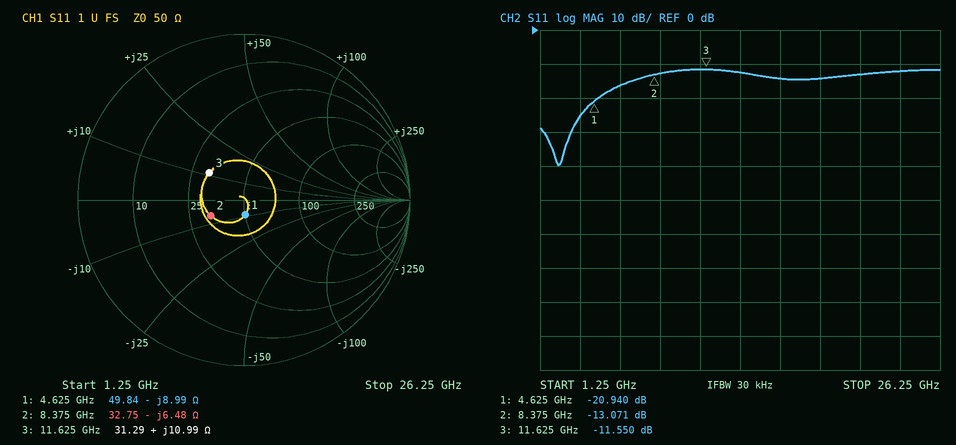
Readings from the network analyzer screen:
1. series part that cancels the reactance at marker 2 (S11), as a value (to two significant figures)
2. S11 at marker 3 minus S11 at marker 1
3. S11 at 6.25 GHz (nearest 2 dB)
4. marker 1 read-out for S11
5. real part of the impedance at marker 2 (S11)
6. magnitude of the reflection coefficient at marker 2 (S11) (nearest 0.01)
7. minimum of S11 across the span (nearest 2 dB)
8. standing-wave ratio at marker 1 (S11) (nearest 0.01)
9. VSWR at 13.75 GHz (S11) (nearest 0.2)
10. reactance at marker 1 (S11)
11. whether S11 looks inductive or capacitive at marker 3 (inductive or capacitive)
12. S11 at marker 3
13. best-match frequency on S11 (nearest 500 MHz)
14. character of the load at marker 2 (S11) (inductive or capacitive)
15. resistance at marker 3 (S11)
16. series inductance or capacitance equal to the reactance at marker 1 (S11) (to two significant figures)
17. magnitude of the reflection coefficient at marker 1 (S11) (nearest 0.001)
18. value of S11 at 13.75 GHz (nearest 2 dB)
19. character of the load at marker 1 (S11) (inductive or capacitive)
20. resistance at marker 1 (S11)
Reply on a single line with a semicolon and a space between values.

120 pH; 9.390 dB; -16 dB; -20.940 dB; 32.75 Ω; 0.22; -40 dB; 1.20; 1.6; -8.99 Ω; inductive; -11.550 dB; 2.5 GHz; capacitive; 31.29 Ω; 3.8 pF; 0.090; -12 dB; capacitive; 49.84 Ω
